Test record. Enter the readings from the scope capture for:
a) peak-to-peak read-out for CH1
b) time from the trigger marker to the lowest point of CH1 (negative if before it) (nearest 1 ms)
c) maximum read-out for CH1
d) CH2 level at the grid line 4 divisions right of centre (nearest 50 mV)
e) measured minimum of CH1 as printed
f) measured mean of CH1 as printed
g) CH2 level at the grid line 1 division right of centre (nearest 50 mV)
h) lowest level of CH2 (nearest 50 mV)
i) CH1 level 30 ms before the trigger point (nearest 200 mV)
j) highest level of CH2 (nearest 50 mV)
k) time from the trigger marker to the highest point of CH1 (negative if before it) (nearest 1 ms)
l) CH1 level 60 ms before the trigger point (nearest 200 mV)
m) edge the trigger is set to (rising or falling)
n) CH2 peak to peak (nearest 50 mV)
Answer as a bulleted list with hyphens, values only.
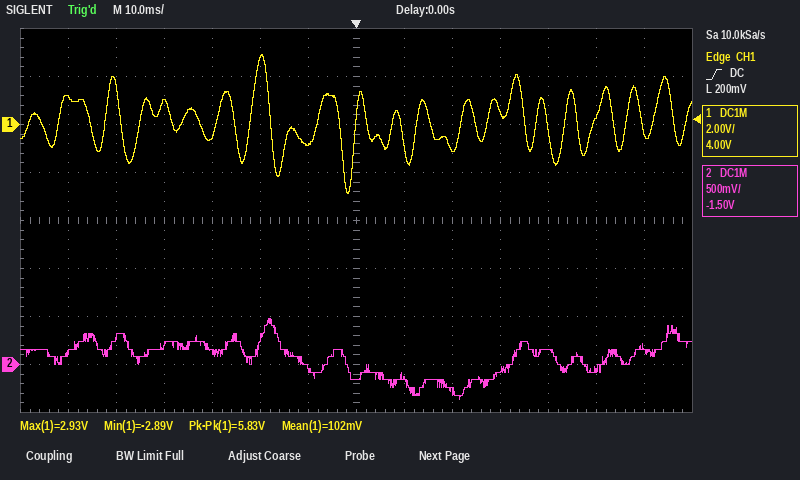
- 5.83 V
- -2 ms
- 2.93 V
- 150 mV
- -2.89 V
- 102 mV
- -150 mV
- -350 mV
- -400 mV
- 500 mV
- -20 ms
- 1.2 V
- rising
- 850 mV
